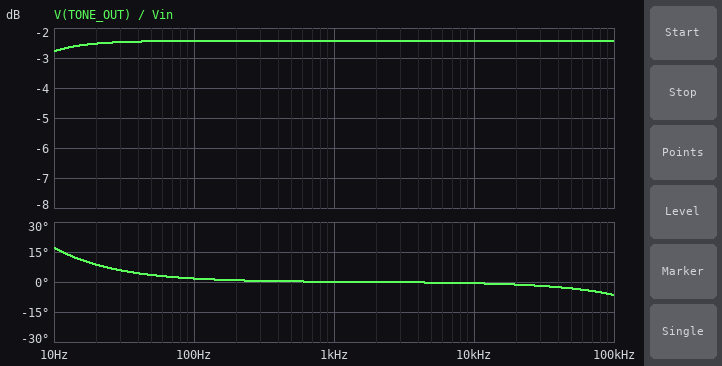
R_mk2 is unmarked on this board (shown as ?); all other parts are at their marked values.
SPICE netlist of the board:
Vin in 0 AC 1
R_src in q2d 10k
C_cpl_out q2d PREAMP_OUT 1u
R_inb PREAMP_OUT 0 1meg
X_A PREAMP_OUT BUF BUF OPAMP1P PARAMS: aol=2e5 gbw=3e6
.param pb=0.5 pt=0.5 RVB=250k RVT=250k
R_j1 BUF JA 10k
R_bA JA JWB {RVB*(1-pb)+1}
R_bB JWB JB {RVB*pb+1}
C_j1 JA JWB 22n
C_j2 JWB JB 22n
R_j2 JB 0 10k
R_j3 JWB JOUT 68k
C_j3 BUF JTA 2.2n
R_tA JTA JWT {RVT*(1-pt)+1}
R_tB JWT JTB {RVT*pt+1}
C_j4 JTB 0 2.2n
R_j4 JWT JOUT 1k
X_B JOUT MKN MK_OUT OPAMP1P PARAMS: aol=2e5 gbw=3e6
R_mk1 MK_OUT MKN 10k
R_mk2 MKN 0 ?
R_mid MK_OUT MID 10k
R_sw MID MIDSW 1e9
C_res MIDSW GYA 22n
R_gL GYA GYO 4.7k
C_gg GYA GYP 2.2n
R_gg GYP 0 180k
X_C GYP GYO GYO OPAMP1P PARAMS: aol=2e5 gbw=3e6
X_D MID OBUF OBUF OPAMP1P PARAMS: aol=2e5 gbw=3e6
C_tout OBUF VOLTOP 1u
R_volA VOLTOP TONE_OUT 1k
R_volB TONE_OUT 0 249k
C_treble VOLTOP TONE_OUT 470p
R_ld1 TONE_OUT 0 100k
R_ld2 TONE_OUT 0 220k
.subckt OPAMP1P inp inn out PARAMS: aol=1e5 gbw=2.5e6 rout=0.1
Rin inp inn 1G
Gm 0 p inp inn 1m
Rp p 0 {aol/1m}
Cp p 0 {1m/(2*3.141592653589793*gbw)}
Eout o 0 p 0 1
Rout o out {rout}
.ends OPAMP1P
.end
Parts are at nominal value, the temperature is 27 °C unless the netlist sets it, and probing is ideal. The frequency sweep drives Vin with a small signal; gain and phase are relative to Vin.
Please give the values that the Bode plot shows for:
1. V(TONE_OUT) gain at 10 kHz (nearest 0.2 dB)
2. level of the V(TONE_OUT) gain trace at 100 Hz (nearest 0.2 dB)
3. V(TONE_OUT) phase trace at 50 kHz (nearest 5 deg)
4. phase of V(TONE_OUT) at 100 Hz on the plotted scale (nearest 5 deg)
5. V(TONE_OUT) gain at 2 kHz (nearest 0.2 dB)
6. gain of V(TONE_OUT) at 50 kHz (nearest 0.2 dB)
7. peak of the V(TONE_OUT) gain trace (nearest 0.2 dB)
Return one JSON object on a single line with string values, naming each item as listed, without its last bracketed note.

{"V(TONE_OUT) gain at 10 kHz": "-2.4 dB", "level of the V(TONE_OUT) gain trace at 100 Hz": "-2.4 dB", "V(TONE_OUT) phase trace at 50 kHz": "-5 deg", "phase of V(TONE_OUT) at 100 Hz on the plotted scale": "0 deg", "V(TONE_OUT) gain at 2 kHz": "-2.4 dB", "gain of V(TONE_OUT) at 50 kHz": "-2.4 dB", "peak of the V(TONE_OUT) gain trace": "-2.4 dB"}
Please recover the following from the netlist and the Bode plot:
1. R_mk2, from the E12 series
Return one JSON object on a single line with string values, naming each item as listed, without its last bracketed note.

{"R_mk2, from the E12 series": "18 kΩ"}
